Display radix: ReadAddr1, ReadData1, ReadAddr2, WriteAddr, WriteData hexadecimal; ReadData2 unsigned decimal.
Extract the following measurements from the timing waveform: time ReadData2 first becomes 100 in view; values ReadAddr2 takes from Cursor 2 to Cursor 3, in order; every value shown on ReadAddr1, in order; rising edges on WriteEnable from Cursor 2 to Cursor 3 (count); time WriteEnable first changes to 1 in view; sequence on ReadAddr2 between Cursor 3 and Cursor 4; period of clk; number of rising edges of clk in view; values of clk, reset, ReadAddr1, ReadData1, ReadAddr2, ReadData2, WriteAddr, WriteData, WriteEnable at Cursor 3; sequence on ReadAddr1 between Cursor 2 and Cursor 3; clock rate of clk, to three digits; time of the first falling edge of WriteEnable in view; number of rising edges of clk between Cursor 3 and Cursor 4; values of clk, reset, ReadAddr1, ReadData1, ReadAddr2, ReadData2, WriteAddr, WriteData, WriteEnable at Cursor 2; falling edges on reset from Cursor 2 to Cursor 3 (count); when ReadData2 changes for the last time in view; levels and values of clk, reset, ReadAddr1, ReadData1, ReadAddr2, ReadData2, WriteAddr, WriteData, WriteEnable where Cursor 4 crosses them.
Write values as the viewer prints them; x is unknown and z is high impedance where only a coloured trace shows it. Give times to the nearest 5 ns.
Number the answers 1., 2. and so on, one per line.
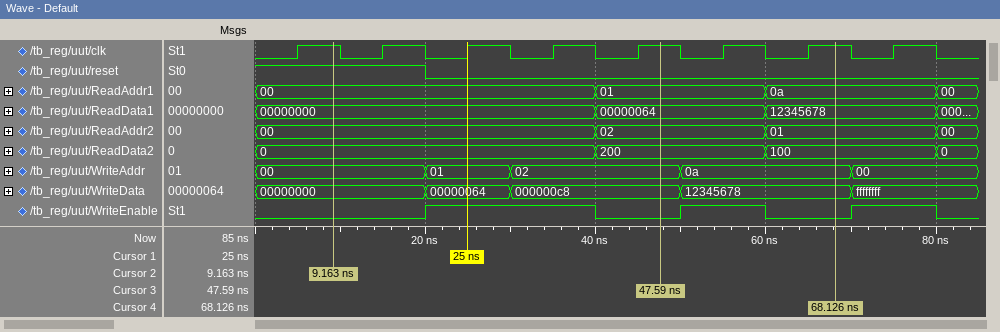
1. 60 ns
2. 00, 02
3. 00, 01, 0a, 00
4. 1
5. 20 ns
6. 02, 01
7. 10 ns
8. 8
9. clk=1, reset=0, ReadAddr1=01, ReadData1=00000064, ReadAddr2=02, ReadData2=200, WriteAddr=02, WriteData=000000c8, WriteEnable=0
10. 00, 01
11. 100 MHz
12. 40 ns
13. 2
14. clk=1, reset=1, ReadAddr1=00, ReadData1=00000000, ReadAddr2=00, ReadData2=0, WriteAddr=00, WriteData=00000000, WriteEnable=0
15. 1
16. 80 ns
17. clk=1, reset=0, ReadAddr1=0a, ReadData1=12345678, ReadAddr2=01, ReadData2=100, WriteAddr=0a, WriteData=12345678, WriteEnable=0
